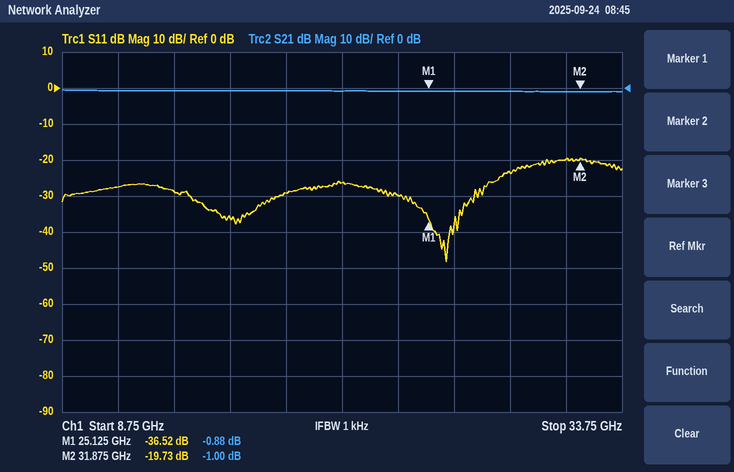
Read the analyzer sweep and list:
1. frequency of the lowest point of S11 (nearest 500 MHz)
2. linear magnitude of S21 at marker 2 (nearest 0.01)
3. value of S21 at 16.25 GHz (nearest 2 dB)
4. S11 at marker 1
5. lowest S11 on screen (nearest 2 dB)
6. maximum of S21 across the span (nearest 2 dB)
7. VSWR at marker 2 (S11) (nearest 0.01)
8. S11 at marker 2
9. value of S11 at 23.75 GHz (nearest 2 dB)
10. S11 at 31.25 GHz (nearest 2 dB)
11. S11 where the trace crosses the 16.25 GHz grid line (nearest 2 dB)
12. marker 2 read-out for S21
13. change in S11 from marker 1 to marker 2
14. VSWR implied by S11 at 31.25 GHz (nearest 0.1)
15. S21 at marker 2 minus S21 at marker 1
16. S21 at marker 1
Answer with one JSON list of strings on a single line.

["26.0 GHz", "0.89", "0 dB", "-36.52 dB", "-48 dB", "0 dB", "1.23", "-19.73 dB", "-30 dB", "-20 dB", "-36 dB", "-1.00 dB", "16.79 dB", "1.2", "-0.12 dB", "-0.88 dB"]
